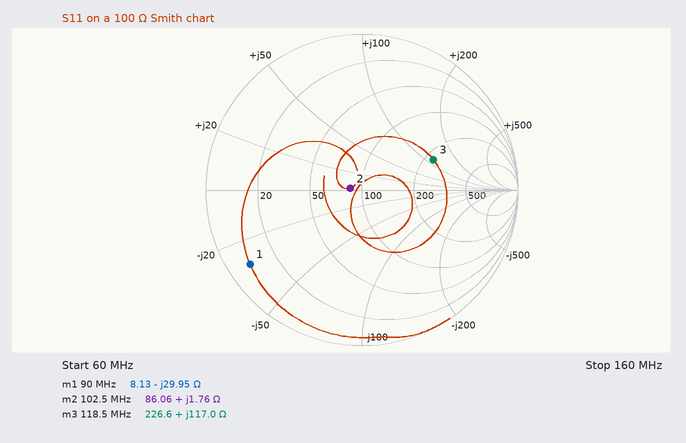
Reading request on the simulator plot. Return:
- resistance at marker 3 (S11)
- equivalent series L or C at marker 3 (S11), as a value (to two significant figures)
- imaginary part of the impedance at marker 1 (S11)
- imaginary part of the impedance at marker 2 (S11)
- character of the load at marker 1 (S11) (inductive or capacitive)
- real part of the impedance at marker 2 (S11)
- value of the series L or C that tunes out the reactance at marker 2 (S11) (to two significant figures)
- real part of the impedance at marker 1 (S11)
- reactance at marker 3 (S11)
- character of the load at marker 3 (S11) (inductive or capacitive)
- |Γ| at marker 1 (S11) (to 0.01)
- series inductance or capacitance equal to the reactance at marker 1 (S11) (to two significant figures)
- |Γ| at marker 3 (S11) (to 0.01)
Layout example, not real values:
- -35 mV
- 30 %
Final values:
- 226.6 Ω
- 160 nH
- -29.95 Ω
- +1.76 Ω
- capacitive
- 86.06 Ω
- 880 pF
- 8.13 Ω
- +117.0 Ω
- inductive
- 0.86
- 59 pF
- 0.50
